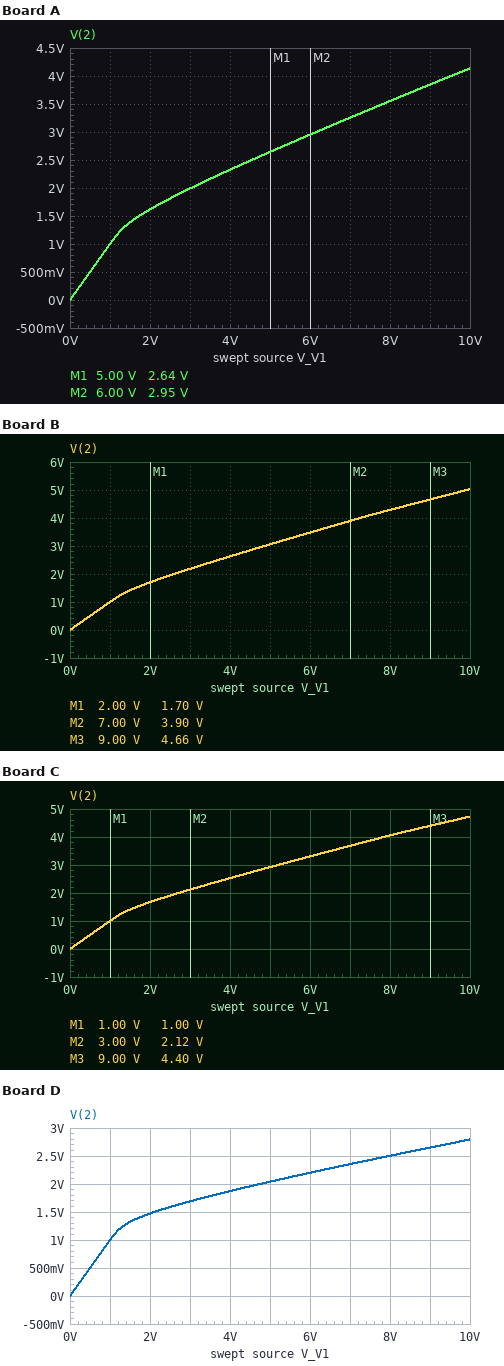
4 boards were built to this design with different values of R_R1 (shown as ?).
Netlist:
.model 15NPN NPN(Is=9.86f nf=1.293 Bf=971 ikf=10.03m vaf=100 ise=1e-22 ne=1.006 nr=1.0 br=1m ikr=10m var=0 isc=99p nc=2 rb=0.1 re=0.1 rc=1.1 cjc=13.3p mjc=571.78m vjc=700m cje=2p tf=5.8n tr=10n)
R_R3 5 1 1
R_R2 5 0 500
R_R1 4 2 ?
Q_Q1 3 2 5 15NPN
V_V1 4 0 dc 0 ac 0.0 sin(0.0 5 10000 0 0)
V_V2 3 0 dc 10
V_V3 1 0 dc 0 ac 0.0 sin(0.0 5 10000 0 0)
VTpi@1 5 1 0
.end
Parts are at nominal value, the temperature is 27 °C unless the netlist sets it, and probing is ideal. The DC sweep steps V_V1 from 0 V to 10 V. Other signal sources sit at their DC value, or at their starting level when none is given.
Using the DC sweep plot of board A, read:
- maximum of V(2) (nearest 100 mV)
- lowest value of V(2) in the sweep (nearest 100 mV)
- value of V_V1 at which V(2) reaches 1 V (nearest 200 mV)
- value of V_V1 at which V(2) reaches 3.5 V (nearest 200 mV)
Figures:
4.1 V
0 V
1.0 V
7.8 V
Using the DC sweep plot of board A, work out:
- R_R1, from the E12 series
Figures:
0.56 Ω
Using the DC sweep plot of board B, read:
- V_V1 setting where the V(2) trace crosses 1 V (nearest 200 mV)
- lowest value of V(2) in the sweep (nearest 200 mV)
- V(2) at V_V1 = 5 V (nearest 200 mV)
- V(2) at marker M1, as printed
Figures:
1.0 V
0 V
3.0 V
1.70 V
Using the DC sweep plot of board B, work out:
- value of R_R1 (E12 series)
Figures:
0.33 Ω
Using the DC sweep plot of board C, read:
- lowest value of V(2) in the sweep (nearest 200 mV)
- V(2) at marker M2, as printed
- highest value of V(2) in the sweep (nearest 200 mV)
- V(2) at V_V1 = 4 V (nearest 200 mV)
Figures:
0 V
2.12 V
4.8 V
2.6 V
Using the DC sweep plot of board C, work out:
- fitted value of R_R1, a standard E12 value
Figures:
0.39 Ω
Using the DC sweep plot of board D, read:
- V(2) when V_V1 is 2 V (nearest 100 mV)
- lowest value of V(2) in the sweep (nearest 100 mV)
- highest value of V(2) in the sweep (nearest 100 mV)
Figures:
1.5 V
0 V
2.8 V
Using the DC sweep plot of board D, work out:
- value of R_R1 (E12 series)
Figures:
1.5 Ω
